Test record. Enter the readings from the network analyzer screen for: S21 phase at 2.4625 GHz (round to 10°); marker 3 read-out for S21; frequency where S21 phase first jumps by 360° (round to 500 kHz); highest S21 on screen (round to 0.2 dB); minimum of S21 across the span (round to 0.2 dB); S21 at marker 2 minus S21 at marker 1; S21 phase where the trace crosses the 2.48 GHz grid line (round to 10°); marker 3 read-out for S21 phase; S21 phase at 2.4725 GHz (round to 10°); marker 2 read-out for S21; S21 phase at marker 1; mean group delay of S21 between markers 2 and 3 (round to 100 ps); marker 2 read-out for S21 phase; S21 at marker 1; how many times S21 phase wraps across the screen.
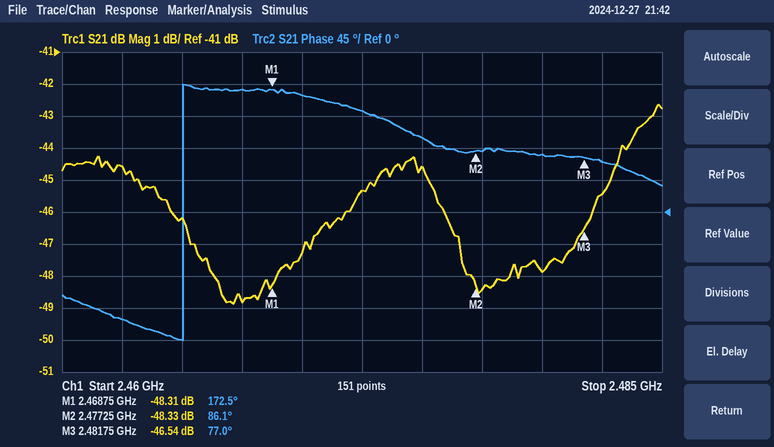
-150°
-46.54 dB
2.4650 GHz
-42.6 dB
-48.8 dB
-0.02 dB
80°
77.0°
140°
-48.33 dB
172.5°
5.6 ns
86.1°
-48.31 dB
1
